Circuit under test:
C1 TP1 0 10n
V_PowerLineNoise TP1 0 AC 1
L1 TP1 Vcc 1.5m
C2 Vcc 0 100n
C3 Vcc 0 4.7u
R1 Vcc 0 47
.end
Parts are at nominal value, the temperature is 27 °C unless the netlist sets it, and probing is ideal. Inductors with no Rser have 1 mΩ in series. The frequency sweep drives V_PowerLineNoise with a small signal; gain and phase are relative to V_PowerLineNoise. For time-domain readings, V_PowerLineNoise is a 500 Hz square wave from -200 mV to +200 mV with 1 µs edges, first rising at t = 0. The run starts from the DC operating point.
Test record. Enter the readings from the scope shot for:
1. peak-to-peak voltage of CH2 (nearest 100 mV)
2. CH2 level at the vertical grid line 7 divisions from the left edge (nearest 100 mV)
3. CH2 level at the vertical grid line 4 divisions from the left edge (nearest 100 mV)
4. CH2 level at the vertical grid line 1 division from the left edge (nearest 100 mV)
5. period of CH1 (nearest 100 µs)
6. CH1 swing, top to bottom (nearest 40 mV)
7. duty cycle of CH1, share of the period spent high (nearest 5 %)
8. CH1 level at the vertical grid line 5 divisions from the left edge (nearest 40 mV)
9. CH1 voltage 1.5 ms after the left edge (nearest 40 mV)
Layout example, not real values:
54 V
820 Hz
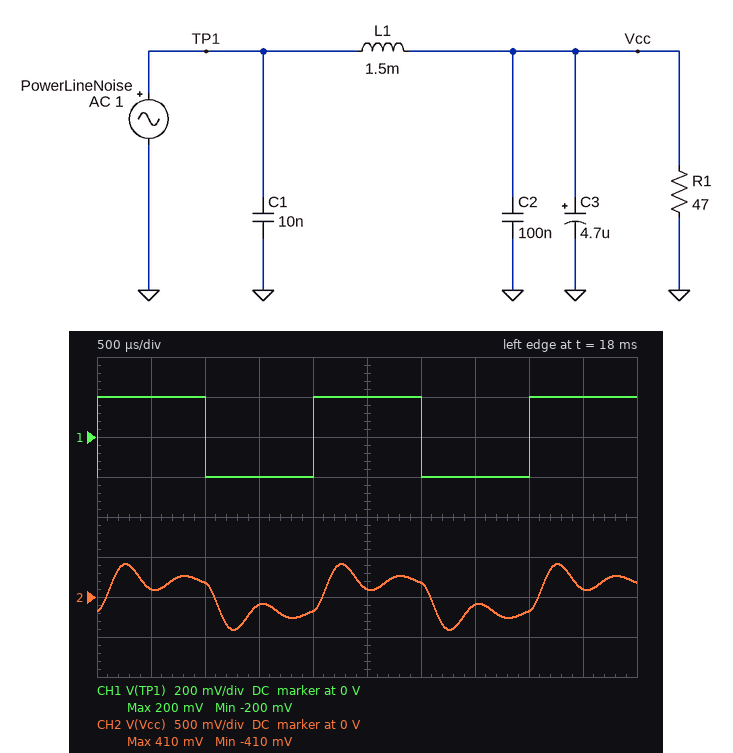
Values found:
800 mV
-100 mV
-200 mV
100 mV
2.0 ms
400 mV
50 %
200 mV
-200 mV
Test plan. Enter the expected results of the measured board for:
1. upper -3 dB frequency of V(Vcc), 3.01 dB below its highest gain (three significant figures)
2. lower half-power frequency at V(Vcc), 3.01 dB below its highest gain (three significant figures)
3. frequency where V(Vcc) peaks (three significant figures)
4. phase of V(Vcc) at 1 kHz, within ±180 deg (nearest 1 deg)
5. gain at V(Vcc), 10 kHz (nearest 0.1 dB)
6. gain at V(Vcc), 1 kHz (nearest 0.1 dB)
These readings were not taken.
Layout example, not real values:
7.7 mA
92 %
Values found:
2.14 kHz
1.40 kHz
1.81 kHz
-16 deg
-28.8 dB
2.6 dB
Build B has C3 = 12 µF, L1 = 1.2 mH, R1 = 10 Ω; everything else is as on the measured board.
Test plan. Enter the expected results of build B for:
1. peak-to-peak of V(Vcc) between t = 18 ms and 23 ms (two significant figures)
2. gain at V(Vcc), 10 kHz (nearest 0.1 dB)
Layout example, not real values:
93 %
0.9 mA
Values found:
530 mV
-35.1 dB
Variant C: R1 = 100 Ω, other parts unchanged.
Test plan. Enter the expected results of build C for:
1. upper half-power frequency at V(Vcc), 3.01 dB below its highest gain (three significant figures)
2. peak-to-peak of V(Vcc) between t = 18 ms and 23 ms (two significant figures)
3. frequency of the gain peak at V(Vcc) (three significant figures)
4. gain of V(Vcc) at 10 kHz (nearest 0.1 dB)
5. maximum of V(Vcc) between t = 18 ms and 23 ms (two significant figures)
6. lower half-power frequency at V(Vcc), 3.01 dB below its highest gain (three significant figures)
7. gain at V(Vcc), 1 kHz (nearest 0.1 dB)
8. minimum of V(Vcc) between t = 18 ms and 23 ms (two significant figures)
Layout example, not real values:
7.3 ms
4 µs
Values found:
2.02 kHz
890 mV
1.86 kHz
-28.8 dB
440 mV
1.69 kHz
2.8 dB
-440 mV
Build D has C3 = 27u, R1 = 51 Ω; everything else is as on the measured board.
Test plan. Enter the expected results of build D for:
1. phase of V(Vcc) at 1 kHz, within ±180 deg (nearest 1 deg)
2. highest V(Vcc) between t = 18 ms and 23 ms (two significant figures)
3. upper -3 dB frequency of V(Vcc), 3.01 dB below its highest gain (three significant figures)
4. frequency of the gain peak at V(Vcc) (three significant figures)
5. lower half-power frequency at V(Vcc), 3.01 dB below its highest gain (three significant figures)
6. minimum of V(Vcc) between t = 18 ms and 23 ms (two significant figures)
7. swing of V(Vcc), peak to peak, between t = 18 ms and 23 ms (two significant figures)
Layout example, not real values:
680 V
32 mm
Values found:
-163 deg
450 mV
841 Hz
785 Hz
725 Hz
-450 mV
890 mV
